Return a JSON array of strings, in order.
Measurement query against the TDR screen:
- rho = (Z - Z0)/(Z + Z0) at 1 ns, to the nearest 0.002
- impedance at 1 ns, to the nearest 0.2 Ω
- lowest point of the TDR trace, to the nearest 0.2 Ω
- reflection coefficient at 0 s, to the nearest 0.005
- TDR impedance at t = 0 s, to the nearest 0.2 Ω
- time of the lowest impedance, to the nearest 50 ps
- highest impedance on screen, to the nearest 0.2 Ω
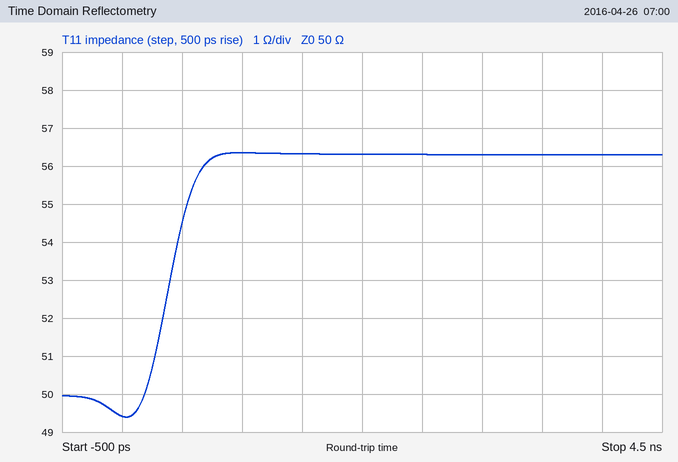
["+0.060", "56.4 Ω", "49.4 Ω", "-0.005", "49.4 Ω", "50 ps", "56.4 Ω"]
